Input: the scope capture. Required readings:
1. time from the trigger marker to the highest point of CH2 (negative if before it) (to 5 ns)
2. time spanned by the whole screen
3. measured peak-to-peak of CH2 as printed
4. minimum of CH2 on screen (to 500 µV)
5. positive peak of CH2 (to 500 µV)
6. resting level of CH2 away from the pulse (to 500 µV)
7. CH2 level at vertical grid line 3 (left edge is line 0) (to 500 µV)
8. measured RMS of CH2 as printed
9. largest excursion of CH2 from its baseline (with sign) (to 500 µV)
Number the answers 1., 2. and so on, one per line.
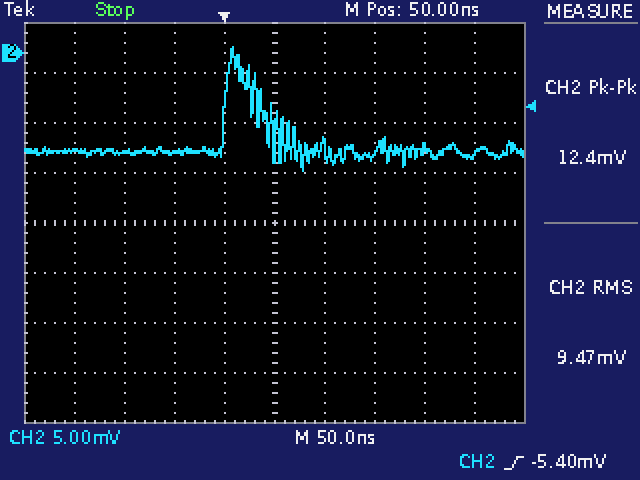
1. +10 ns
2. 500 ns
3. 12.4 mV
4. -12.0 mV
5. 500 µV
6. -10.0 mV
7. -10.0 mV
8. 9.47 mV
9. +10.5 mV
